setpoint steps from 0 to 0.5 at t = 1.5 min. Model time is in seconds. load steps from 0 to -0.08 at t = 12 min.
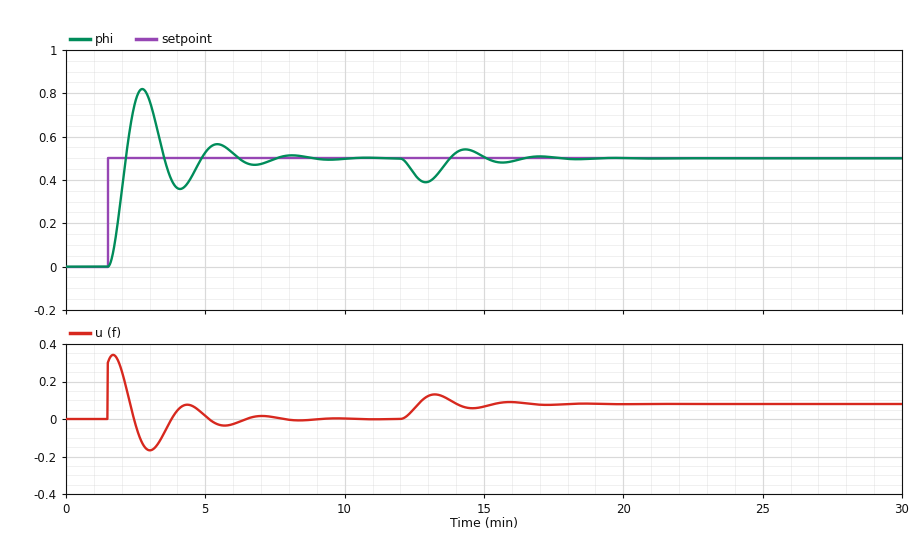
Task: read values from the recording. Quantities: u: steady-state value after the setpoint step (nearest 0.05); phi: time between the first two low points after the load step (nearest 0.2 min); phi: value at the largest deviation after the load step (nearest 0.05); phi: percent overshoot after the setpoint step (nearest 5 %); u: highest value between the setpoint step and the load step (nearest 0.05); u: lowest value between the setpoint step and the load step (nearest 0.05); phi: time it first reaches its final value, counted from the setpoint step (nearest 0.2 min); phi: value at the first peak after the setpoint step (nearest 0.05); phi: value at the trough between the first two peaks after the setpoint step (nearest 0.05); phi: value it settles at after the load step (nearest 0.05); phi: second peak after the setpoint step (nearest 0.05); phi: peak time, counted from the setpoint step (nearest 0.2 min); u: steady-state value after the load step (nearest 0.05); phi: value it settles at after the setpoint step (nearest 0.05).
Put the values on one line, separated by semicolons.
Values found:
0.00; 2.8 min; 0.40; 65 %; 0.35; -0.15; 0.6 min; 0.80; 0.35; 0.50; 0.55; 1.2 min; 0.10; 0.50
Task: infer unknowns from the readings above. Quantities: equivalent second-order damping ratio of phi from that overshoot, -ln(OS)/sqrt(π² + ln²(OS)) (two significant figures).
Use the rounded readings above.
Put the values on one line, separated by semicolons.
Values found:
0.14
